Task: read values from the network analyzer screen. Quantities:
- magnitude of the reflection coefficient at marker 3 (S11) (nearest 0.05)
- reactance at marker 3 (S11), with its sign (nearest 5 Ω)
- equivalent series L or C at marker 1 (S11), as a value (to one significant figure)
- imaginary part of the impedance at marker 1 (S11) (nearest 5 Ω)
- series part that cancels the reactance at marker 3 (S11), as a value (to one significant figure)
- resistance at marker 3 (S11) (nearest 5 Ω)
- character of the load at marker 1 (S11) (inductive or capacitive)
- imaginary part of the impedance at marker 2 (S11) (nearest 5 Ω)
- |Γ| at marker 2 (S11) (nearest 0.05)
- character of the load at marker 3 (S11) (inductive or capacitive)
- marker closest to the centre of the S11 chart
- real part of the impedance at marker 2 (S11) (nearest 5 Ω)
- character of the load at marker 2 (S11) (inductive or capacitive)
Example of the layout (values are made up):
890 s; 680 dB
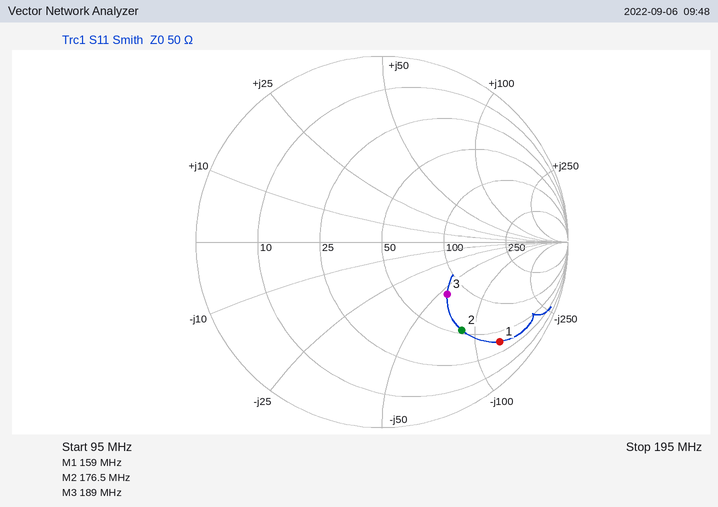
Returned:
0.45; -55 Ω; 8 pF; -125 Ω; 50 nH; 80 Ω; capacitive; -85 Ω; 0.65; capacitive; marker 3; 55 Ω; capacitive
